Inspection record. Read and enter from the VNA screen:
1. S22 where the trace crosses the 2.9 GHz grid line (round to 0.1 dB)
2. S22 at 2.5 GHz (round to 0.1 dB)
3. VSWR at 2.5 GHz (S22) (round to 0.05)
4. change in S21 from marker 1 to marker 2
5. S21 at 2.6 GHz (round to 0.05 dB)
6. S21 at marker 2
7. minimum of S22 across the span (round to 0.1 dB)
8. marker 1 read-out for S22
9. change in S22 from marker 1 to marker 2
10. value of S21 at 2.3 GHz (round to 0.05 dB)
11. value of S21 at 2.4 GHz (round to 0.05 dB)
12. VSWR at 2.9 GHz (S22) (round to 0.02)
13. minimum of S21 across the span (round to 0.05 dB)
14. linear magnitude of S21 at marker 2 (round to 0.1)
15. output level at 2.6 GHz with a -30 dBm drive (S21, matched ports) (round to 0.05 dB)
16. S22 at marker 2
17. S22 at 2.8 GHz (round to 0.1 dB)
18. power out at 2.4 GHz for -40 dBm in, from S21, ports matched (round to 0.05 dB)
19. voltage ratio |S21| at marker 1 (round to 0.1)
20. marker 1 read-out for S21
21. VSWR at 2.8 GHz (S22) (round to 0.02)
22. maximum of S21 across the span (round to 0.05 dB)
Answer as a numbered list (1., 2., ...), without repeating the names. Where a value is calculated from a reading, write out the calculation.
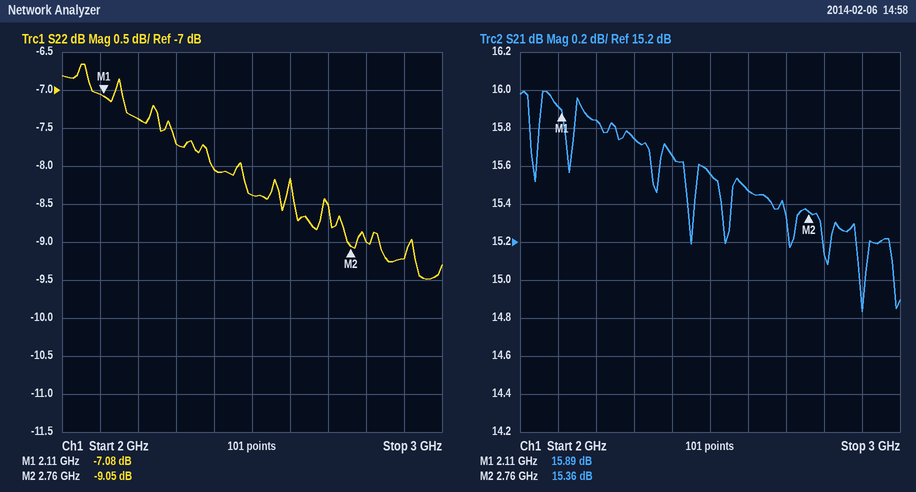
1. -9.2 dB
2. -8.4 dB
3. |Γ| = 10^(-8.4/20) = 0.3802; VSWR = (1 + 0.3802)/(1 − 0.3802) ≈ 2.23, so 2.25 to the nearest 0.05
4. 15.36 − (15.89) = -0.53 dB
5. 15.45 dB
6. 15.36 dB
7. -9.5 dB
8. -7.08 dB
9. -9.05 − (-7.08) = -1.97 dB
10. 15.75 dB
11. 15.65 dB
12. |Γ| = 10^(-9.2/20) = 0.3467; VSWR = (1 + 0.3467)/(1 − 0.3467) ≈ 2.06
13. 14.85 dB
14. 10^(15.36/20) ≈ 5.9
15. -30 dBm + (15.45 dB) = -14.55 dBm
16. -9.05 dB
17. -9.0 dB
18. -40 dBm + (15.65 dB) = -24.35 dBm
19. 10^(15.89/20) ≈ 6.2
20. 15.89 dB
21. |Γ| = 10^(-9/20) = 0.3548; VSWR = (1 + 0.3548)/(1 − 0.3548) ≈ 2.10
22. 16.00 dB
